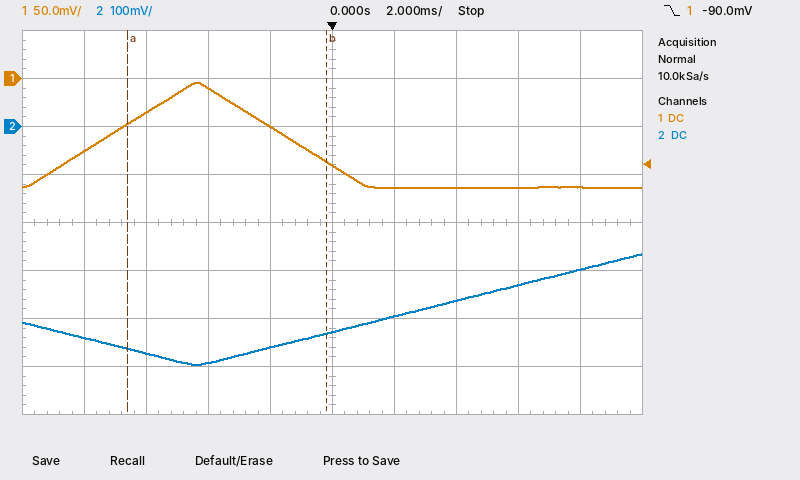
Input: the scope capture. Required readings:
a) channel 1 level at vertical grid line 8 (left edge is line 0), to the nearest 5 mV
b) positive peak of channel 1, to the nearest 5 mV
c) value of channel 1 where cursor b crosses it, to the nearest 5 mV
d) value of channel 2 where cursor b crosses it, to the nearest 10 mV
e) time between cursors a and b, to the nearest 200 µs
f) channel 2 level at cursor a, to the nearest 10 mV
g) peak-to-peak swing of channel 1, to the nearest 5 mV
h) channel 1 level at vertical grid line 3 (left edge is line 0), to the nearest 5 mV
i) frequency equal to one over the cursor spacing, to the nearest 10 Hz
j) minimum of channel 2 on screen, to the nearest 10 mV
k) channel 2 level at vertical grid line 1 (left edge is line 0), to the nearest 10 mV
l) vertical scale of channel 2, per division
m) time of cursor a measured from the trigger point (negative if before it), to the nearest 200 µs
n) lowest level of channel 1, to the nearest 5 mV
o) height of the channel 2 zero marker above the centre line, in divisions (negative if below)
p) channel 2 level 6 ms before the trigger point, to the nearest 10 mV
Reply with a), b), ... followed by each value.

a) -115 mV
b) -5 mV
c) -85 mV
d) -430 mV
e) 6.4 ms
f) -460 mV
g) 110 mV
h) -10 mV
i) 160 Hz
j) -500 mV
k) -440 mV
l) 100 mV
m) -6.6 ms
n) -115 mV
o) +2.0 div
p) -470 mV
